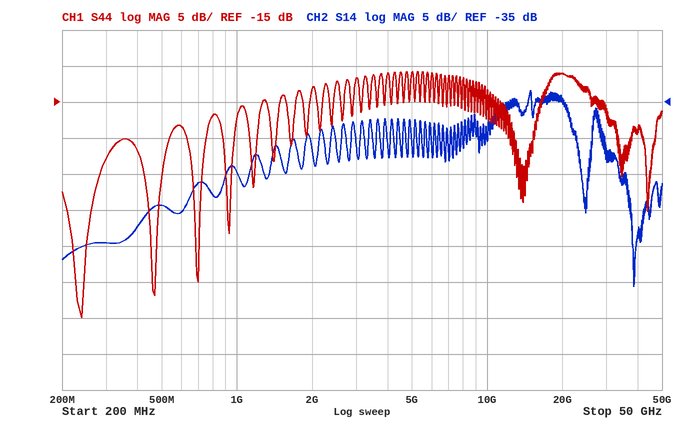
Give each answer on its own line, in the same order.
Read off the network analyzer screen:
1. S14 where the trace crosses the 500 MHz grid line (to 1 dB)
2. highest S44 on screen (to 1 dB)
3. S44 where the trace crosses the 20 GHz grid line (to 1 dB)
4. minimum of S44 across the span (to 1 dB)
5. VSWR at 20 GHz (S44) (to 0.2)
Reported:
-49 dB
-11 dB
-11 dB
-45 dB
1.8
